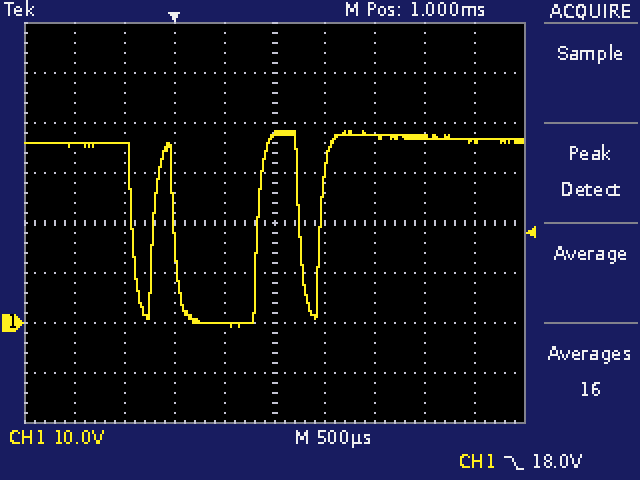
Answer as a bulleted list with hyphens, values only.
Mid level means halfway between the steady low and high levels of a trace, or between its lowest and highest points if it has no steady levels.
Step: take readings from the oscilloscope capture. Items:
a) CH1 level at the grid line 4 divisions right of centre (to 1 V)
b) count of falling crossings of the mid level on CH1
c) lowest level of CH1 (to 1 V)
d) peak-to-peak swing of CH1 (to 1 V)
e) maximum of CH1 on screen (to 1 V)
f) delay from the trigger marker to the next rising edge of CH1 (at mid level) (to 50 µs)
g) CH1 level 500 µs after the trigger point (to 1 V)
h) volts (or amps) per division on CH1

- 36 V
- 3
- -1 V
- 39 V
- 38 V
- 850 µs
- 0 V
- 10 V
